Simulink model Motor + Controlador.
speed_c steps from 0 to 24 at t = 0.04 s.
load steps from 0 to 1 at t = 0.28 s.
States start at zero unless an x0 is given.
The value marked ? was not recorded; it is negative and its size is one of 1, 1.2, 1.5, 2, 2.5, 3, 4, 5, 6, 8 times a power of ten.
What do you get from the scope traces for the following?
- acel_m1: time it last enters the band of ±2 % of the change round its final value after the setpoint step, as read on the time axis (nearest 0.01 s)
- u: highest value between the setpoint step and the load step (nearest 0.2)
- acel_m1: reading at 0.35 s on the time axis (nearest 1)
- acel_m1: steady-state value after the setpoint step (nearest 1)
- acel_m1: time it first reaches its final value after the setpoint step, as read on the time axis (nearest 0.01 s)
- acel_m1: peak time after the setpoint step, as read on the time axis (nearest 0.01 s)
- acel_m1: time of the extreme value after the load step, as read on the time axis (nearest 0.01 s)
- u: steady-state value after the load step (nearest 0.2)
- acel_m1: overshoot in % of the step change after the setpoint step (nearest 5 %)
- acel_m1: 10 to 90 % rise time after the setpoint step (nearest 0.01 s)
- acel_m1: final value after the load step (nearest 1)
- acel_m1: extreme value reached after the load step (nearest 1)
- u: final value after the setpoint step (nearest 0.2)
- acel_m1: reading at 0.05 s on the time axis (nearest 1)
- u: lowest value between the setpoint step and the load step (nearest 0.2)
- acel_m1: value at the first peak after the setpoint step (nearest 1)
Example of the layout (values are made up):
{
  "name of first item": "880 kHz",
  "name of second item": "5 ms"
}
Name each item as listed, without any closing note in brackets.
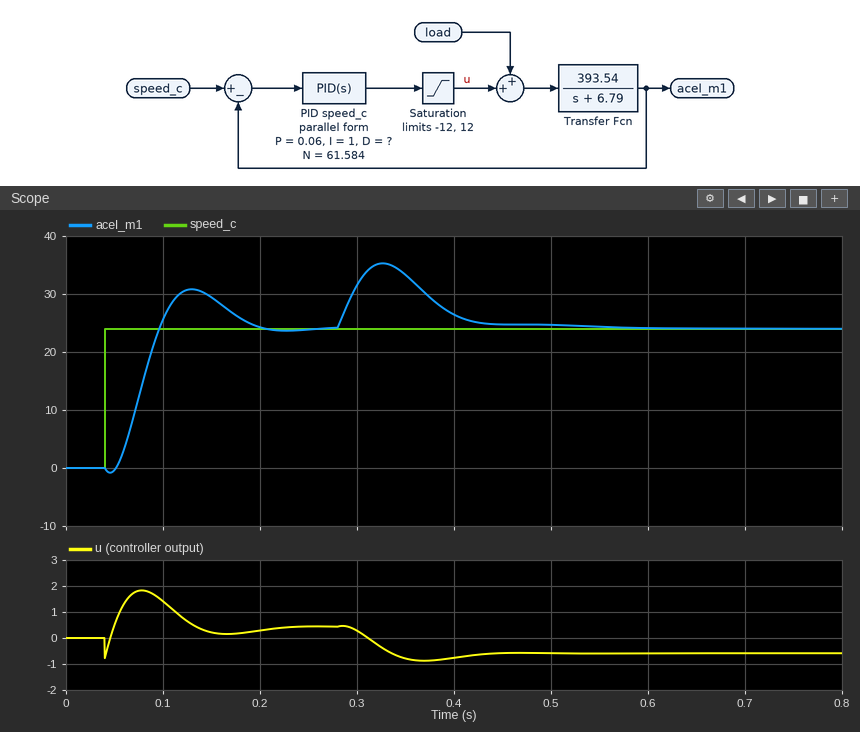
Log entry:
{
  "acel_m1: time it last enters the band of ±2 % of the change round its final value after the setpoint step, as read on the time axis": "0.20 s",
  "u: highest value between the setpoint step and the load step": "1.8",
  "acel_m1: reading at 0.35 s on the time axis": "33",
  "acel_m1: steady-state value after the setpoint step": "24",
  "acel_m1: time it first reaches its final value after the setpoint step, as read on the time axis": "0.10 s",
  "acel_m1: peak time after the setpoint step, as read on the time axis": "0.13 s",
  "acel_m1: time of the extreme value after the load step, as read on the time axis": "0.33 s",
  "u: steady-state value after the load step": "-0.6",
  "acel_m1: overshoot in % of the step change after the setpoint step": "30 %",
  "acel_m1: 10 to 90 % rise time after the setpoint step": "0.03 s",
  "acel_m1: final value after the load step": "24",
  "acel_m1: extreme value reached after the load step": "35",
  "u: final value after the setpoint step": "0.4",
  "acel_m1: reading at 0.05 s on the time axis": "0",
  "u: lowest value between the setpoint step and the load step": "-0.8",
  "acel_m1: value at the first peak after the setpoint step": "31"
}
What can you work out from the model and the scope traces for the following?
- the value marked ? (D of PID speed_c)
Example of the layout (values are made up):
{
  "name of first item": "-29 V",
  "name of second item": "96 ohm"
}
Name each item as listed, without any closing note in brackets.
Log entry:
{
  "the value marked ?": "-0.0015"
}
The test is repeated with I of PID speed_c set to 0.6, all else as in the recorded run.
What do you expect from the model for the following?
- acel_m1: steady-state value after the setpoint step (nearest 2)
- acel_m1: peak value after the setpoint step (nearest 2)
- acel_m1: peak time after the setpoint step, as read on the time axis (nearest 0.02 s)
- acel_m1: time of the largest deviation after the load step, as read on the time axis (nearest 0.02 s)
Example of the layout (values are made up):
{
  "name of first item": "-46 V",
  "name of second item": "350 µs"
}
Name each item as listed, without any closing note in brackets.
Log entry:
{
  "acel_m1: steady-state value after the setpoint step": "24",
  "acel_m1: peak value after the setpoint step": "28",
  "acel_m1: peak time after the setpoint step, as read on the time axis": "0.14 s",
  "acel_m1: time of the largest deviation after the load step, as read on the time axis": "0.34 s"
}
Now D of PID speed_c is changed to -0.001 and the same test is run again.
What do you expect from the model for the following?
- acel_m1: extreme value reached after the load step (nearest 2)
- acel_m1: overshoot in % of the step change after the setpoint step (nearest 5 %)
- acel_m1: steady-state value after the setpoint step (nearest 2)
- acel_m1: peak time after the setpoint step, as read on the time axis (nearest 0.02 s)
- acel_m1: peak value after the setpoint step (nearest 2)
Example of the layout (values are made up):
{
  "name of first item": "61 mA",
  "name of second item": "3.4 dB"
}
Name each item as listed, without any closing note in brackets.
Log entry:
{
  "acel_m1: extreme value reached after the load step": "34",
  "acel_m1: overshoot in % of the step change after the setpoint step": "20 %",
  "acel_m1: steady-state value after the setpoint step": "24",
  "acel_m1: peak time after the setpoint step, as read on the time axis": "0.14 s",
  "acel_m1: peak value after the setpoint step": "28"
}
